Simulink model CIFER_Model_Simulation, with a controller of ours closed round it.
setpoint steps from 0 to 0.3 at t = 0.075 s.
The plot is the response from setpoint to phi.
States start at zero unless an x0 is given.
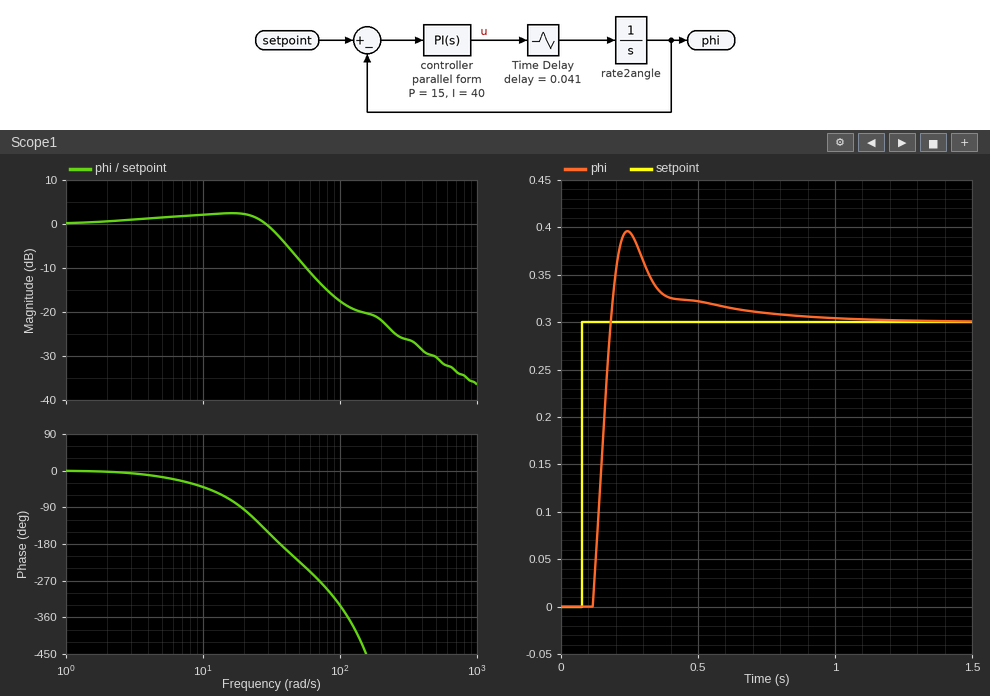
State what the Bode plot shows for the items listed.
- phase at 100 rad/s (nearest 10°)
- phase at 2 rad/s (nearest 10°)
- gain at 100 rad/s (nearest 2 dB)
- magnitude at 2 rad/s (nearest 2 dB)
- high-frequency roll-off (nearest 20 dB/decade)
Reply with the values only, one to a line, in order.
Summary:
-330°
0°
-18 dB
0 dB
-20 dB/decade
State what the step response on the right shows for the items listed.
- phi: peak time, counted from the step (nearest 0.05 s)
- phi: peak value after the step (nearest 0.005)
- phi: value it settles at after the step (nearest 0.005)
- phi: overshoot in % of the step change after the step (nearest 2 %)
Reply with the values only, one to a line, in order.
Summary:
0.15 s
0.395
0.300
32 %
